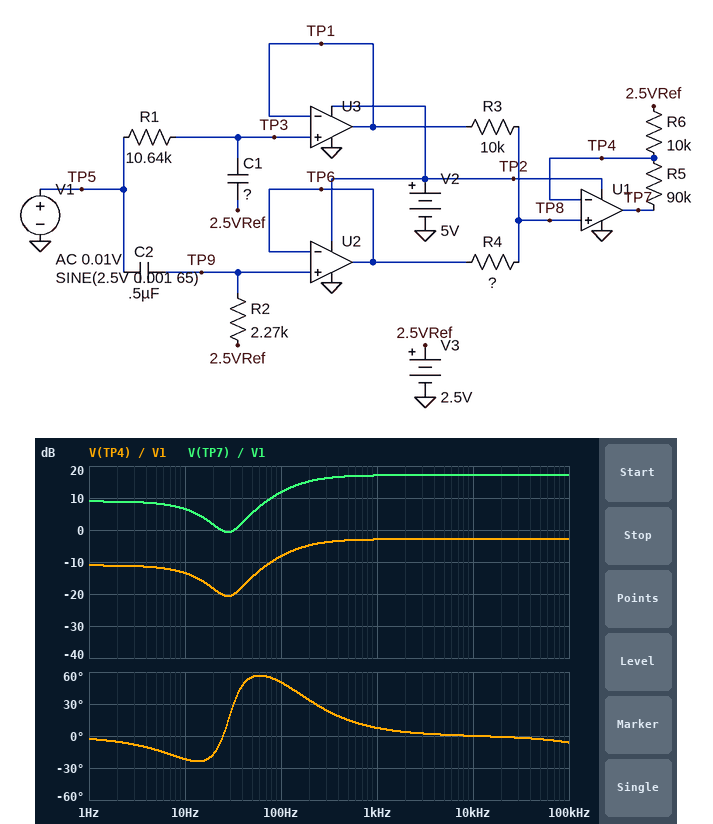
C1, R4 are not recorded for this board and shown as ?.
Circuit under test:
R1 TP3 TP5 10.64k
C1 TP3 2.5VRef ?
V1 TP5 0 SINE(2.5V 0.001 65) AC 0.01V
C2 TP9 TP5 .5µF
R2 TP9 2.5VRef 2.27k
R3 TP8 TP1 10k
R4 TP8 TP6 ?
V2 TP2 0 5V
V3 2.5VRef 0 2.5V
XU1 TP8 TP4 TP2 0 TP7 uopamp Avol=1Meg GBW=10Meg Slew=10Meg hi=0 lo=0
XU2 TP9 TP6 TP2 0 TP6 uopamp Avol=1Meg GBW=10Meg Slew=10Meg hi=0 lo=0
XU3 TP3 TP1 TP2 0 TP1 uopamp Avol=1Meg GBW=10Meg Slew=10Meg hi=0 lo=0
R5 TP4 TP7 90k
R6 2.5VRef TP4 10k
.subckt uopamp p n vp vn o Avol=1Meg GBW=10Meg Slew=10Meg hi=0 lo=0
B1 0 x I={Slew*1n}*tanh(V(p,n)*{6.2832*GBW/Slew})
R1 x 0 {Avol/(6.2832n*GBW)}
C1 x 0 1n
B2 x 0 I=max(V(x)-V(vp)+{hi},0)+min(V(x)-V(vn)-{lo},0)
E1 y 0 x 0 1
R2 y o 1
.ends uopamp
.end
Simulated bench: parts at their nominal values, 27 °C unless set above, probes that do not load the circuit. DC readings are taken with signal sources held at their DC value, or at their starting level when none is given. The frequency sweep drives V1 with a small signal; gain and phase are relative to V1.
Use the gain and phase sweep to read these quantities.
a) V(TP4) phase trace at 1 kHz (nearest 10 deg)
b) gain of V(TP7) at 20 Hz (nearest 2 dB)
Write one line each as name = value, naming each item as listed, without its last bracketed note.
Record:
V(TP4) phase trace at 1 kHz = 10 deg
gain of V(TP7) at 20 Hz = 2 dB
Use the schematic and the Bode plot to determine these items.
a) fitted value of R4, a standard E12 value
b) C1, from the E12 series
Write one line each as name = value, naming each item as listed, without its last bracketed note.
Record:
fitted value of R4, a standard E12 value = 3.9 kΩ
C1, from the E12 series = 1 µF
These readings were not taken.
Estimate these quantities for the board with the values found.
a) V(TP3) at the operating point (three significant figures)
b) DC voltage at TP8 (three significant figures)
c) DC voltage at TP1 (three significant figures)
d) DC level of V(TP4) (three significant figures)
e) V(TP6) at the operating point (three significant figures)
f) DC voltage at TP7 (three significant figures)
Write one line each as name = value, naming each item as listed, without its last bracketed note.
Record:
V(TP3) at the operating point = 2.50 V
DC voltage at TP8 = 2.50 V
DC voltage at TP1 = 2.50 V
DC level of V(TP4) = 2.50 V
V(TP6) at the operating point = 2.50 V
DC voltage at TP7 = 2.50 V
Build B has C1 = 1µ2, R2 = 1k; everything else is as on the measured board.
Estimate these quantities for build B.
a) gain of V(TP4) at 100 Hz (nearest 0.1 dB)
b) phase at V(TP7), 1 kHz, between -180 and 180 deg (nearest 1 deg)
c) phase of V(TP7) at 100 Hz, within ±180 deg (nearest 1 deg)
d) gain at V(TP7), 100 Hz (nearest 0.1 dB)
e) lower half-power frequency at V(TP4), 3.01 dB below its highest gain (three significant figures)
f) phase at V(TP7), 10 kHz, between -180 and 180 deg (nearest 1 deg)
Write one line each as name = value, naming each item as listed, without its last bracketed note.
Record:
gain of V(TP4) at 100 Hz = -14.7 dB
phase at V(TP7), 1 kHz, between -180 and 180 deg = 17 deg
phase of V(TP7) at 100 Hz, within ±180 deg = 68 deg
gain at V(TP7), 100 Hz = 5.3 dB
lower half-power frequency at V(TP4), 3.01 dB below its highest gain = 327 Hz
phase at V(TP7), 10 kHz, between -180 and 180 deg = 1 deg
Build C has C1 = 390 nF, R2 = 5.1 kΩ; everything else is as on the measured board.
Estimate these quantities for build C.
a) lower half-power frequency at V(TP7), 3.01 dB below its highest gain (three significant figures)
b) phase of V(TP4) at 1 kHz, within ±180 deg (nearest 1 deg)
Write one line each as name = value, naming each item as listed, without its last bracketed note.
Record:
lower half-power frequency at V(TP7), 3.01 dB below its highest gain = 65.8 Hz
phase of V(TP4) at 1 kHz, within ±180 deg = 3 deg
